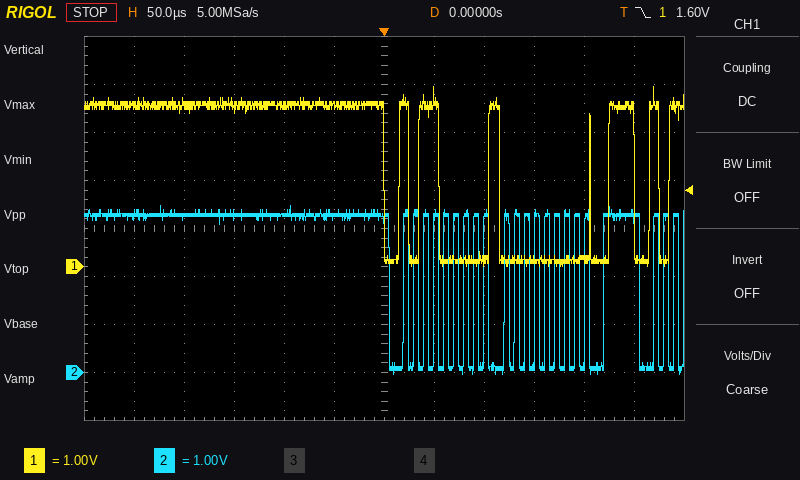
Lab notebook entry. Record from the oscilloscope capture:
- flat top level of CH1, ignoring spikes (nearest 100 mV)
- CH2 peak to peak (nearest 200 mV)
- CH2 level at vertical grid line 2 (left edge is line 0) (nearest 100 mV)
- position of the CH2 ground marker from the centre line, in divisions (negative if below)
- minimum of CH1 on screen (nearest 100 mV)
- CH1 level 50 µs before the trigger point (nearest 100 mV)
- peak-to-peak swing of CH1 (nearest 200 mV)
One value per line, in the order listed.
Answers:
3.4 V
3.6 V
3.2 V
-3.0 div
0.0 V
3.4 V
3.8 V
